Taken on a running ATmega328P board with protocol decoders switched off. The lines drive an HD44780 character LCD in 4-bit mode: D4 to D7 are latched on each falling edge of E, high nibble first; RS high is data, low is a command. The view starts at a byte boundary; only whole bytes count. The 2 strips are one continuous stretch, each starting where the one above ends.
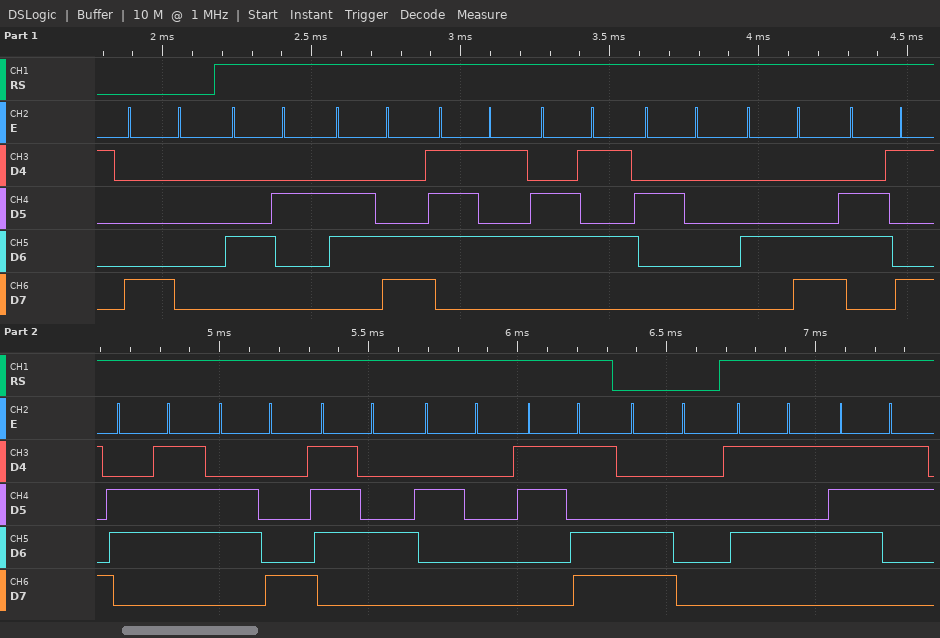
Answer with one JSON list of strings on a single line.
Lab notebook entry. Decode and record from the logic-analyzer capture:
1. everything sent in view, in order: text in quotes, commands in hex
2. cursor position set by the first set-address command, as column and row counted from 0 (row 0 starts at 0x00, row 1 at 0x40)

["0x80 \"Blue Light =\" 0xC0 \"Us\"", "column 0, row 0"]
